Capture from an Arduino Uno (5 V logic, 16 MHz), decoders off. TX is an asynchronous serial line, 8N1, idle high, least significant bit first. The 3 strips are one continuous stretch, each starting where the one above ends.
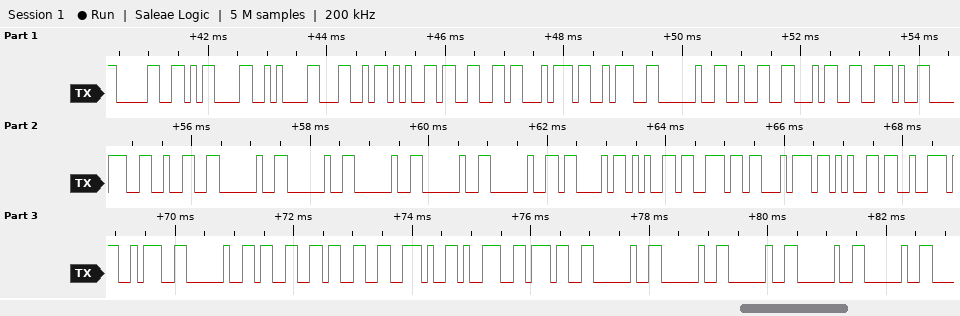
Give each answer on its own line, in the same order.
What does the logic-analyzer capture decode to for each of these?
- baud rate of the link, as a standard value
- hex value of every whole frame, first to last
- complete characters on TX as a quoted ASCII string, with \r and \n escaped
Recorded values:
9600 baud
30 0D 0A 4C 65 66 74 3A 20 32 34 2E 38 32 20 20 20 20 20 43 65 6E 74 65 72 3A 20 33 33 2E 39 37 20 20 20 20 20
"0\r\nLeft: 24.82     Center: 33.97     "
